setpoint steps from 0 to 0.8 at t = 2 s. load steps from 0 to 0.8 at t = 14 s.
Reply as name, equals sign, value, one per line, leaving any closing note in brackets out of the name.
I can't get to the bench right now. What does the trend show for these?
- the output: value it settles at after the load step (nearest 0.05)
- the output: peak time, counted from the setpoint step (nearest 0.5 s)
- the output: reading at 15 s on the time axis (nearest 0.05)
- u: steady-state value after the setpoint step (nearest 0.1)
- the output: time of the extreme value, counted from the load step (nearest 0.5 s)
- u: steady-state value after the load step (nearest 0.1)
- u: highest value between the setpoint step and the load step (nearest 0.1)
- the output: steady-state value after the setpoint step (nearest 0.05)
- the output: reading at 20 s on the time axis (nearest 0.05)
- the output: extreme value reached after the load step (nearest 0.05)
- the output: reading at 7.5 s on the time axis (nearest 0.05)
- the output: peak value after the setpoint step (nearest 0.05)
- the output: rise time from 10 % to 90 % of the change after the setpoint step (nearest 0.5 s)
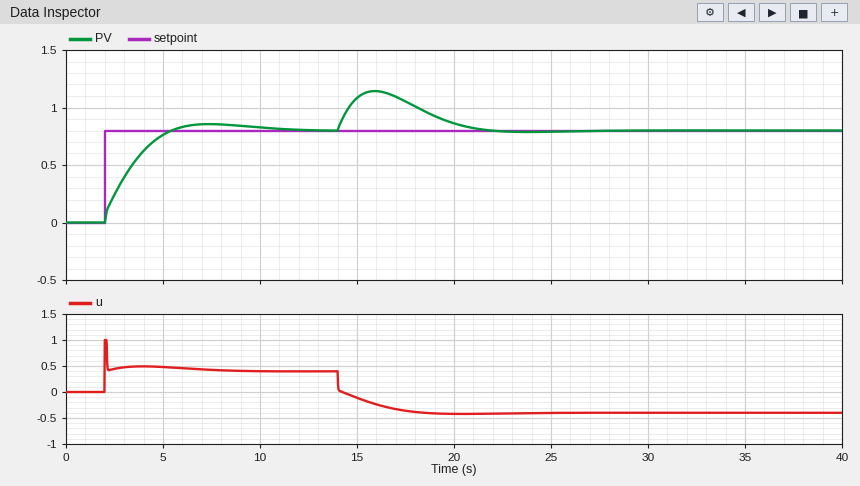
the output: value it settles at after the load step = 0.80
the output: peak time, counted from the setpoint step = 5.5 s
the output: reading at 15 s on the time axis = 1.10
u: steady-state value after the setpoint step = 0.4
the output: time of the extreme value, counted from the load step = 2.0 s
u: steady-state value after the load step = -0.4
u: highest value between the setpoint step and the load step = 1.0
the output: steady-state value after the setpoint step = 0.80
the output: reading at 20 s on the time axis = 0.85
the output: extreme value reached after the load step = 1.15
the output: reading at 7.5 s on the time axis = 0.85
the output: peak value after the setpoint step = 0.85
the output: rise time from 10 % to 90 % of the change after the setpoint step = 2.5 s
